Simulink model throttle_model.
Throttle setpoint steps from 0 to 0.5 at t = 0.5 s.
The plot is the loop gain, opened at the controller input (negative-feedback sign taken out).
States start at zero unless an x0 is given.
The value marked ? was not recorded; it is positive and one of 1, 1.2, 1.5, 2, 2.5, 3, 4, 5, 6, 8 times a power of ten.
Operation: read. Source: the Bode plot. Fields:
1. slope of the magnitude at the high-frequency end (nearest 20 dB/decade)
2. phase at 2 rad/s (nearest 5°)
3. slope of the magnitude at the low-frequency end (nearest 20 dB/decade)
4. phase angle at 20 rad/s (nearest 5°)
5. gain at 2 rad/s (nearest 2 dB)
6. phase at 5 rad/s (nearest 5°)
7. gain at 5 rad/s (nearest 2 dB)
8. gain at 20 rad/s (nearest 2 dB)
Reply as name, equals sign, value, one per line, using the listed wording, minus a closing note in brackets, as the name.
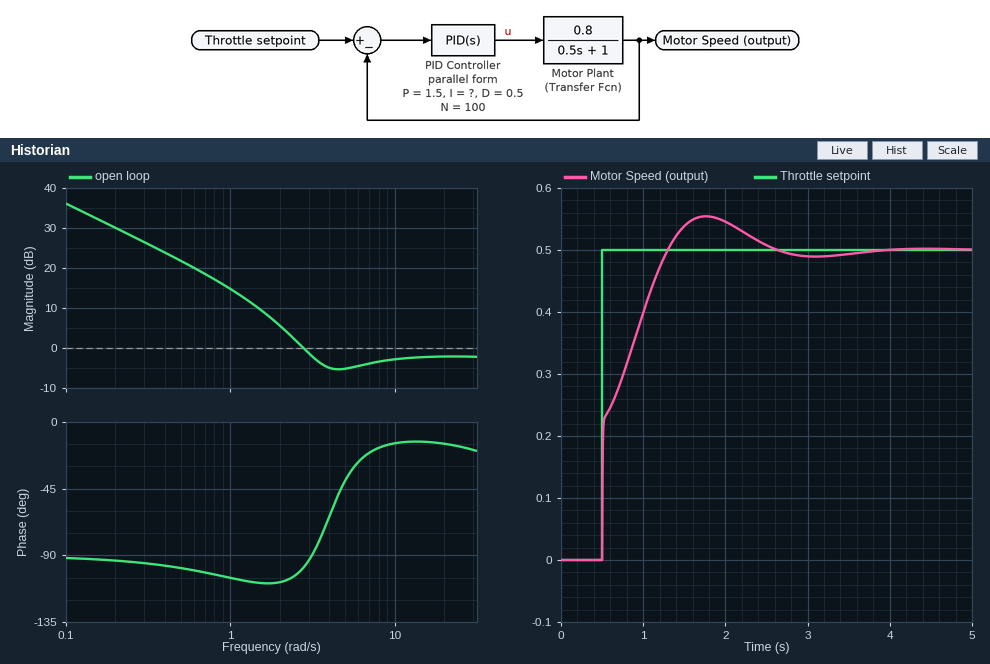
slope of the magnitude at the high-frequency end = 0 dB/decade
phase at 2 rad/s = -110°
slope of the magnitude at the low-frequency end = -20 dB/decade
phase angle at 20 rad/s = -15°
gain at 2 rad/s = 6 dB
phase at 5 rad/s = -40°
gain at 5 rad/s = -6 dB
gain at 20 rad/s = -2 dB
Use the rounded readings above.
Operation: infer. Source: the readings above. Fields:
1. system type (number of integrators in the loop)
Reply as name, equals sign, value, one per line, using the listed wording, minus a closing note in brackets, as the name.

system type = 1
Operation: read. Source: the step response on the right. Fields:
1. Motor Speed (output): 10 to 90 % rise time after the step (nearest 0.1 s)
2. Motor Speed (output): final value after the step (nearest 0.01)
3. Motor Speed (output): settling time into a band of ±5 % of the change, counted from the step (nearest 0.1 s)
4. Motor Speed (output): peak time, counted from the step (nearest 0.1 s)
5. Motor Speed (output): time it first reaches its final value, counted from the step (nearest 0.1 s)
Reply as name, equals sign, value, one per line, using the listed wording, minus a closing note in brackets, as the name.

Motor Speed (output): 10 to 90 % rise time after the step = 0.6 s
Motor Speed (output): final value after the step = 0.50
Motor Speed (output): settling time into a band of ±5 % of the change, counted from the step = 1.8 s
Motor Speed (output): peak time, counted from the step = 1.3 s
Motor Speed (output): time it first reaches its final value, counted from the step = 0.8 s
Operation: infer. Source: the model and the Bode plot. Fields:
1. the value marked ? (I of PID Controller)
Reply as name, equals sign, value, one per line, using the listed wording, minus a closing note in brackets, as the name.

the value marked ? = 8
